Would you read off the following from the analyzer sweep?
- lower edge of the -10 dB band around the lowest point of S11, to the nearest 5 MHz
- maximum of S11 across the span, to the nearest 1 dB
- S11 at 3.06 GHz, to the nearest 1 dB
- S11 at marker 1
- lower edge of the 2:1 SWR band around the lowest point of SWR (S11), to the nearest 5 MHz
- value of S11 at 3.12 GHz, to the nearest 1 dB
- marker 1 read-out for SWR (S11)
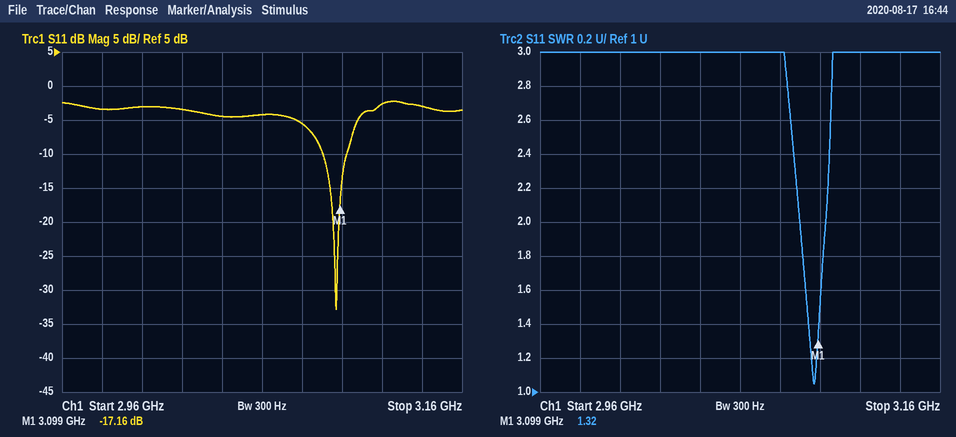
3.090 GHz
-2 dB
-4 dB
-17.16 dB
3.090 GHz
-3 dB
1.32
